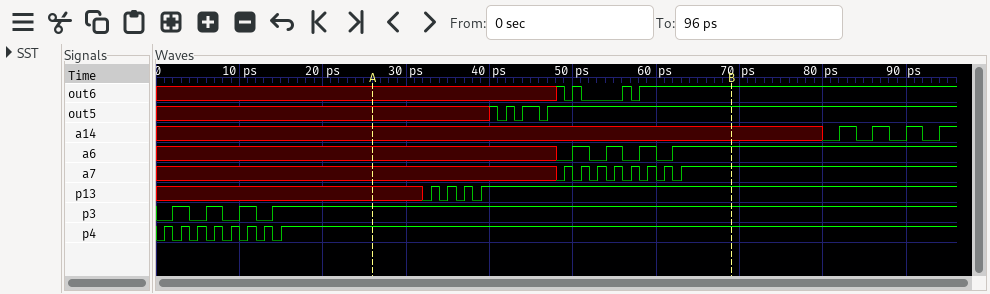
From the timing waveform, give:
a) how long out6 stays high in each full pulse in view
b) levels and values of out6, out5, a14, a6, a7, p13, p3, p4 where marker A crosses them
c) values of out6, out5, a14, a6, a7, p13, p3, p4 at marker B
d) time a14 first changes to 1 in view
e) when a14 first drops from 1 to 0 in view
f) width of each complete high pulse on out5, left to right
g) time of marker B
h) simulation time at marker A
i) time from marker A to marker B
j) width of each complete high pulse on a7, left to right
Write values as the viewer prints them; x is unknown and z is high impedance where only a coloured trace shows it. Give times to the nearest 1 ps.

1 ps, 1 ps
out6=x, out5=x, a14=x, a6=x, a7=x, p13=x, p3=1, p4=1
out6=1, out5=1, a14=x, a6=1, a7=1, p13=1, p3=1, p4=1
82 ps
84 ps
1 ps, 2 ps
69 ps
26 ps
43 ps
1 ps, 1 ps, 1 ps, 1 ps, 1 ps, 1 ps, 1 ps
